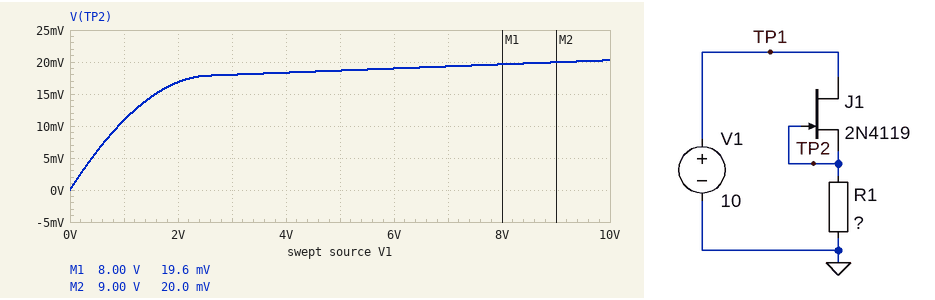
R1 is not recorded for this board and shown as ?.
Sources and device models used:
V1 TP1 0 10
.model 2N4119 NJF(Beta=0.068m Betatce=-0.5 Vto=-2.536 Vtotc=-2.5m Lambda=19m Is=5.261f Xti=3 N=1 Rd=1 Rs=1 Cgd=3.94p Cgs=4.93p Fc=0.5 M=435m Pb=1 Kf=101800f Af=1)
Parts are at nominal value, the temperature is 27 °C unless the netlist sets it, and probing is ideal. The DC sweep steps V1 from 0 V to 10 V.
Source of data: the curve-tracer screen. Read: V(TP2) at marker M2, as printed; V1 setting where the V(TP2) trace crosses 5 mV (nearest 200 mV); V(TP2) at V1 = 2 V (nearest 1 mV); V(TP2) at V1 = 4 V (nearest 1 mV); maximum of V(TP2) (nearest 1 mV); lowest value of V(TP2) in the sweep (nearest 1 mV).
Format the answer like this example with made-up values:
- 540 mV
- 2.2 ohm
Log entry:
- 20.0 mV
- 400 mV
- 17 mV
- 18 mV
- 20 mV
- 0 V
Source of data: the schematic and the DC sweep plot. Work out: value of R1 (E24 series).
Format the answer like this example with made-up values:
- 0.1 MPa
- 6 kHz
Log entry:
- 39 Ω
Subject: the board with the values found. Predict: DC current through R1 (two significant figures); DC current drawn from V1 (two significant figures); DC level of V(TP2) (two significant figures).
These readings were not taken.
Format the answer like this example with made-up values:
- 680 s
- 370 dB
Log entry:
- 520 µA
- 520 µA
- 20 mV
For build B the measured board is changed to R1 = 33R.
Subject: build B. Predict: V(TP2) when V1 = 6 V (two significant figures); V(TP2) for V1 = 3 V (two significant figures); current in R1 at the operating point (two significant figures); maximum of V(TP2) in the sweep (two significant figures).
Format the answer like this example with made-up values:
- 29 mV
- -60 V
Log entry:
- 16 mV
- 15 mV
- 520 µA
- 17 mV
